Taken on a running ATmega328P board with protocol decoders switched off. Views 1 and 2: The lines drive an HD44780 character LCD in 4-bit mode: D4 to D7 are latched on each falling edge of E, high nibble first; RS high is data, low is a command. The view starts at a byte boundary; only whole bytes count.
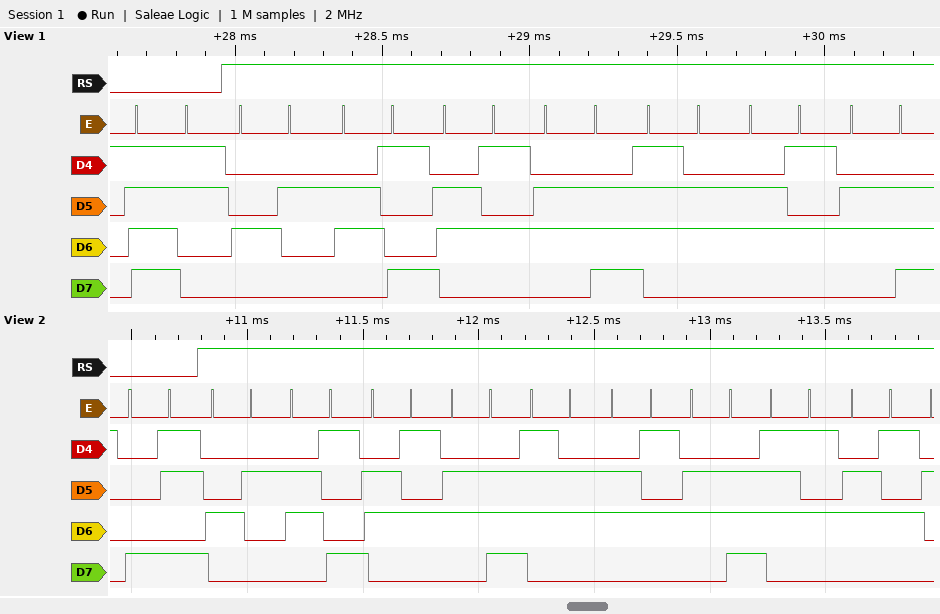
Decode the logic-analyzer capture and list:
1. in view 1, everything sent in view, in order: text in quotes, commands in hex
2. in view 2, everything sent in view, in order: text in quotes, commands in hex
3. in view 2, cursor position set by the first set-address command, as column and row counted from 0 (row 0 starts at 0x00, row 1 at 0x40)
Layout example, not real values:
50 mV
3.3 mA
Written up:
0xF3 "Bienven"
0x8B "Bienvenue"
column 11, row 0
